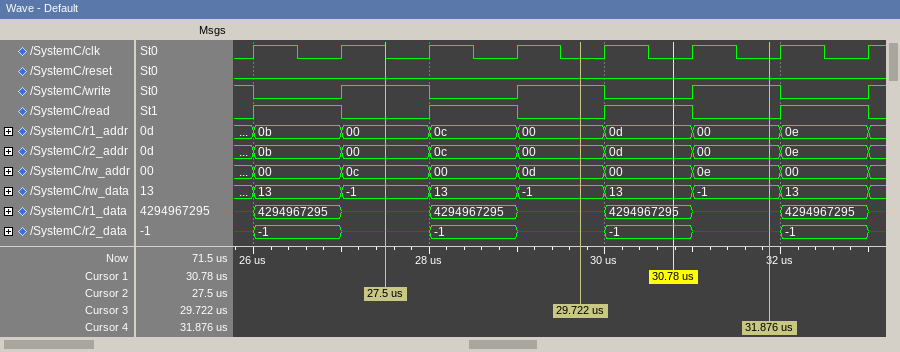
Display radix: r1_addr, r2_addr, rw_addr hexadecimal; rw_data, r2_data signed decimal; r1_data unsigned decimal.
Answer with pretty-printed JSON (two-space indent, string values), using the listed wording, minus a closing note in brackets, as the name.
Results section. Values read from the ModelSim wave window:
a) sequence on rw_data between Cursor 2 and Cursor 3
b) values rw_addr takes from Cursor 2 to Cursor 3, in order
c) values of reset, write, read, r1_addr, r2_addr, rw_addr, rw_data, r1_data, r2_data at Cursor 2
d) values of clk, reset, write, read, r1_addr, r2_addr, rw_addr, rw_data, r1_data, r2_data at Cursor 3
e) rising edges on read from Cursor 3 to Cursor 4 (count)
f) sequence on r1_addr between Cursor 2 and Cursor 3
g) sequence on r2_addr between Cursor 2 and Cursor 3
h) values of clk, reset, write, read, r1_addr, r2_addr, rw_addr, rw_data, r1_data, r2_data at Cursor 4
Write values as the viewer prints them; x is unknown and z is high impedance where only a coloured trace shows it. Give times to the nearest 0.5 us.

{
  "sequence on rw_data between Cursor 2 and Cursor 3": "-1, 13, -1",
  "values rw_addr takes from Cursor 2 to Cursor 3, in order": "0c, 00, 0d",
  "values of reset, write, read, r1_addr, r2_addr, rw_addr, rw_data, r1_data, r2_data at Cursor 2": "reset=0, write=1, read=0, r1_addr=00, r2_addr=00, rw_addr=0c, rw_data=-1, r1_data=x, r2_data=x",
  "values of clk, reset, write, read, r1_addr, r2_addr, rw_addr, rw_data, r1_data, r2_data at Cursor 3": "clk=0, reset=0, write=1, read=0, r1_addr=00, r2_addr=00, rw_addr=0d, rw_data=-1, r1_data=x, r2_data=x",
  "rising edges on read from Cursor 3 to Cursor 4": "1",
  "sequence on r1_addr between Cursor 2 and Cursor 3": "00, 0c, 00",
  "sequence on r2_addr between Cursor 2 and Cursor 3": "00, 0c, 00",
  "values of clk, reset, write, read, r1_addr, r2_addr, rw_addr, rw_data, r1_data, r2_data at Cursor 4": "clk=0, reset=0, write=1, read=0, r1_addr=00, r2_addr=00, rw_addr=0e, rw_data=-1, r1_data=x, r2_data=x"
}
